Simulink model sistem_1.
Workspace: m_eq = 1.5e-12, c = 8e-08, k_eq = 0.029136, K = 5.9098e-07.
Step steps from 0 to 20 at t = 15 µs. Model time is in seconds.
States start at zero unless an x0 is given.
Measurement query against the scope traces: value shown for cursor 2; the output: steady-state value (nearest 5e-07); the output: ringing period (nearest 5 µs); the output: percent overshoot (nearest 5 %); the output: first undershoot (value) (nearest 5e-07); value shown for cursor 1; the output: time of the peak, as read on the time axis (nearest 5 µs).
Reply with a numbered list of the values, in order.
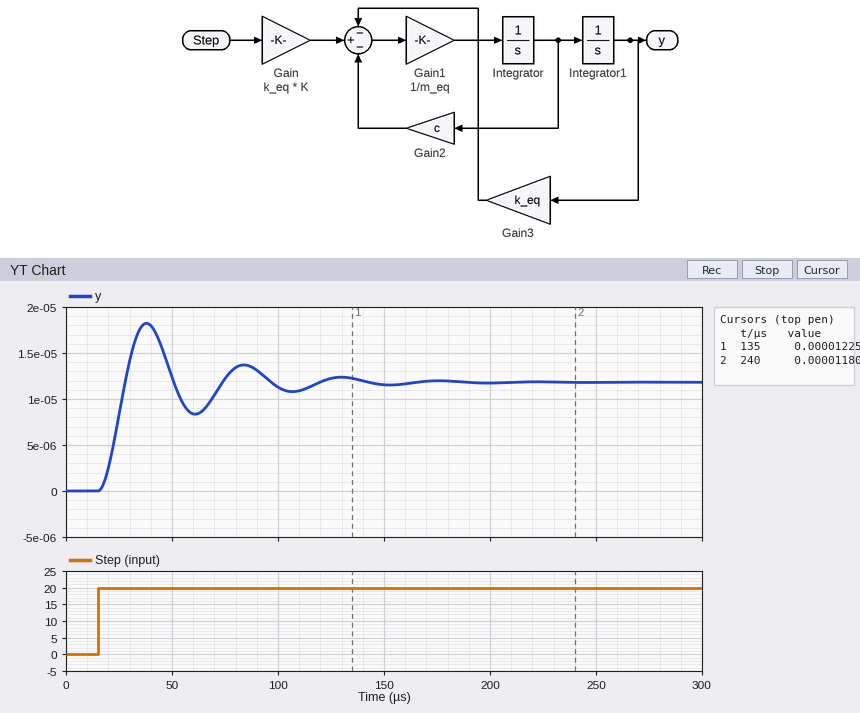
1. 0.00001180
2. 0.0000120
3. 45 µs
4. 55 %
5. 0.0000085
6. 0.00001225
7. 40 µs
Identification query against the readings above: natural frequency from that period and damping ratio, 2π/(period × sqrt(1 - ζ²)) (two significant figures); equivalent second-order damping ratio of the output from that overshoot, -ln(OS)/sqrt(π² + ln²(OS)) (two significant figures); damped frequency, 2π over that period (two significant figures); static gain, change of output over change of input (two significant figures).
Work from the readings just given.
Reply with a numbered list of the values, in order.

1. 0.14 rad/µs
2. 0.19
3. 0.14 rad/µs
4. 0.00000060
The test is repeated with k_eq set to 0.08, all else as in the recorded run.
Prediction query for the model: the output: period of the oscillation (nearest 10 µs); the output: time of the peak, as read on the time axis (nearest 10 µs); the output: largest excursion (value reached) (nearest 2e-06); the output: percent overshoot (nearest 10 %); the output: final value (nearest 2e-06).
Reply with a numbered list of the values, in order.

1. 30 µs
2. 30 µs
3. 0.000020
4. 70 %
5. 0.000012
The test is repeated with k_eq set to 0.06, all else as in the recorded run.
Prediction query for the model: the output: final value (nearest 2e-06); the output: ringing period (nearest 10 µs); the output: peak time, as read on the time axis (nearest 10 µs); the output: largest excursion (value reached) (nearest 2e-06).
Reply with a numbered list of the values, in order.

1. 0.000012
2. 30 µs
3. 30 µs
4. 0.000020
